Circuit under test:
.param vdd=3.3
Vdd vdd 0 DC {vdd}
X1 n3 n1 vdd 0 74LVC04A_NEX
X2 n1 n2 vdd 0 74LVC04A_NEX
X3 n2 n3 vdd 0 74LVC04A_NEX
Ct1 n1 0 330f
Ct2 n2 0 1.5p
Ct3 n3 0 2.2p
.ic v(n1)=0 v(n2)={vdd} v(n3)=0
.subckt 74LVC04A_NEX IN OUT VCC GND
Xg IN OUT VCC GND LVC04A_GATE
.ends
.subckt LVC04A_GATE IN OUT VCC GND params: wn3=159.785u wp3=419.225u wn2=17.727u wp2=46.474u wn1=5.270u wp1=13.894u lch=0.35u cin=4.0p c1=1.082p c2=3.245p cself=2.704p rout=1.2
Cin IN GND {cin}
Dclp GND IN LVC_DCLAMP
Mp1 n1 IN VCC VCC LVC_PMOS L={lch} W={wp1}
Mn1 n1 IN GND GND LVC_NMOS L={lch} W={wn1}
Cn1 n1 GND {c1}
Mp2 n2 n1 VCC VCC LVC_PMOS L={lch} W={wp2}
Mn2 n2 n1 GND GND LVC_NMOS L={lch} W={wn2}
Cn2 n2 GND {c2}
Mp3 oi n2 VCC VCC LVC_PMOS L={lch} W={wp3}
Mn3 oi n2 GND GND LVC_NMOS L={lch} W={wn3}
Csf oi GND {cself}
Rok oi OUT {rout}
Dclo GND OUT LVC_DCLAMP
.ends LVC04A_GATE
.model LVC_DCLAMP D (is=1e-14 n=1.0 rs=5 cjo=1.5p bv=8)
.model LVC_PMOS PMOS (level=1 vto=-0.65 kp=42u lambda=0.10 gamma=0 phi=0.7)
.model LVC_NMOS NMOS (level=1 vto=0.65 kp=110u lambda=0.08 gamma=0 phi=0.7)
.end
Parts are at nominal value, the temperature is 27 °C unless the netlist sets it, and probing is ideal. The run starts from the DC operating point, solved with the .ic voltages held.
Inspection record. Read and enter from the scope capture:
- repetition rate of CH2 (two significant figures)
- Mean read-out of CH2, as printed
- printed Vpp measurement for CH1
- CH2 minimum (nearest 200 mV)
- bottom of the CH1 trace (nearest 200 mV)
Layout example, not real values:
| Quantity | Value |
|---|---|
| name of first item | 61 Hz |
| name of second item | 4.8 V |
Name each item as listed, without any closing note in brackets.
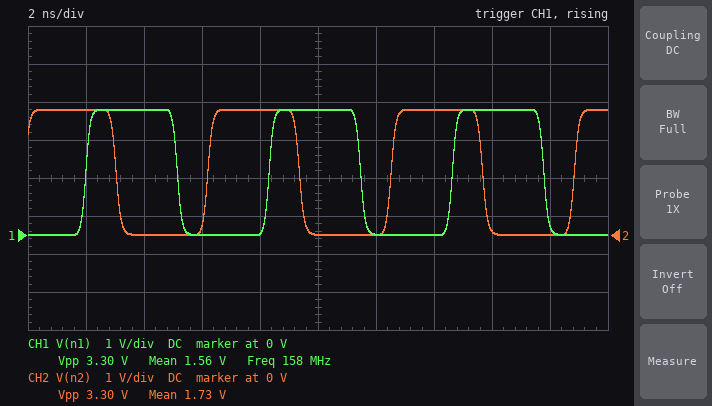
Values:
| Quantity | Value |
|---|---|
| repetition rate of CH2 | 160 MHz |
| Mean read-out of CH2, as printed | 1.73 V |
| printed Vpp measurement for CH1 | 3.30 V |
| CH2 minimum | 0 V |
| bottom of the CH1 trace | 0 V |
